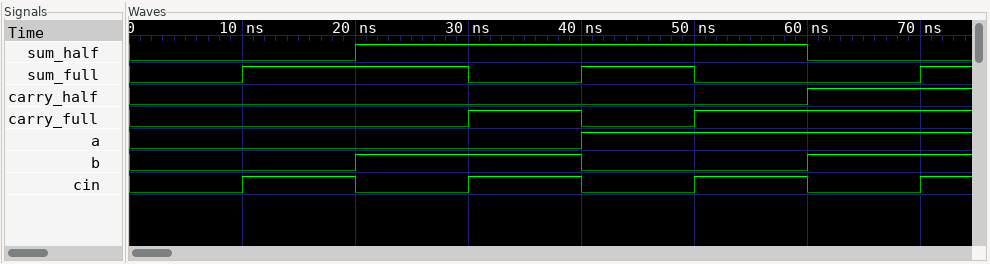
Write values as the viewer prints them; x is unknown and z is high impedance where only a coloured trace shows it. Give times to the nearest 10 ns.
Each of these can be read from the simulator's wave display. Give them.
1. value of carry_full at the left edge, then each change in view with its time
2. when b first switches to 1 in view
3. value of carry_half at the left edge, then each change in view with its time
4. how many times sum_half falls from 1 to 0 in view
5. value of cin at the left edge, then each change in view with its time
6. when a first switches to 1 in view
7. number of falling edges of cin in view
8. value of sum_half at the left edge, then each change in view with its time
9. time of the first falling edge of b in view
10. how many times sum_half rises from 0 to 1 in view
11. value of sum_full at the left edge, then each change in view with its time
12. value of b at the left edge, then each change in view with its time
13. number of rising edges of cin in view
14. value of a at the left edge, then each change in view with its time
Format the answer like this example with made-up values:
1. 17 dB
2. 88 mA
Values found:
1. 0, 1 at 30 ns, 0 at 40 ns, 1 at 50 ns
2. 20 ns
3. 0, 1 at 60 ns
4. 1
5. 0, 1 at 10 ns, 0 at 20 ns, 1 at 30 ns, 0 at 40 ns, 1 at 50 ns, 0 at 60 ns, 1 at 70 ns
6. 40 ns
7. 3
8. 0, 1 at 20 ns, 0 at 60 ns
9. 40 ns
10. 1
11. 0, 1 at 10 ns, 0 at 30 ns, 1 at 40 ns, 0 at 50 ns, 1 at 70 ns
12. 0, 1 at 20 ns, 0 at 40 ns, 1 at 60 ns
13. 4
14. 0, 1 at 40 ns
